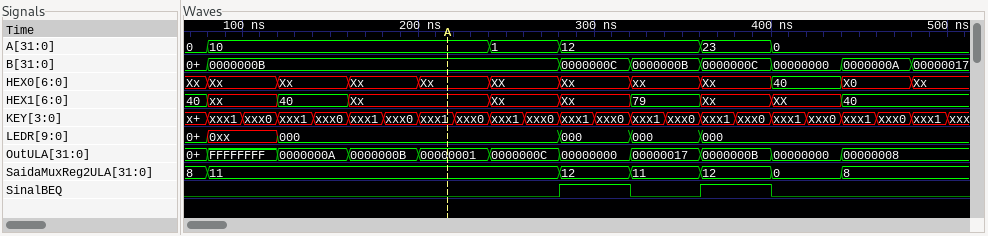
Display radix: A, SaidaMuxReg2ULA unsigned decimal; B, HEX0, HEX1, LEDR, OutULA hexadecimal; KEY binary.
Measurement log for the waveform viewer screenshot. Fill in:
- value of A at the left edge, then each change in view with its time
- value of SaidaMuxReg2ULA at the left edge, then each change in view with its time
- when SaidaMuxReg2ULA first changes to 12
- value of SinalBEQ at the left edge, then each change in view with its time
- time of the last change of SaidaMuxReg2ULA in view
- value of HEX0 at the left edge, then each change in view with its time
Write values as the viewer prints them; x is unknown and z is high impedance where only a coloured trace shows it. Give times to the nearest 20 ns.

0, 10 at 80 ns, 1 at 240 ns, 12 at 280 ns, 23 at 360 ns, 0 at 400 ns
8, 11 at 80 ns, 12 at 280 ns, 11 at 320 ns, 12 at 360 ns, 0 at 400 ns, 8 at 440 ns
280 ns
0, 1 at 280 ns, 0 at 320 ns, 1 at 360 ns, 0 at 400 ns
440 ns
Xx, Xx at 80 ns, Xx at 120 ns, Xx at 160 ns, Xx at 200 ns, XX at 240 ns, Xx at 280 ns, xx at 320 ns, Xx at 360 ns, 40 at 400 ns, X0 at 440 ns, Xx at 480 ns
